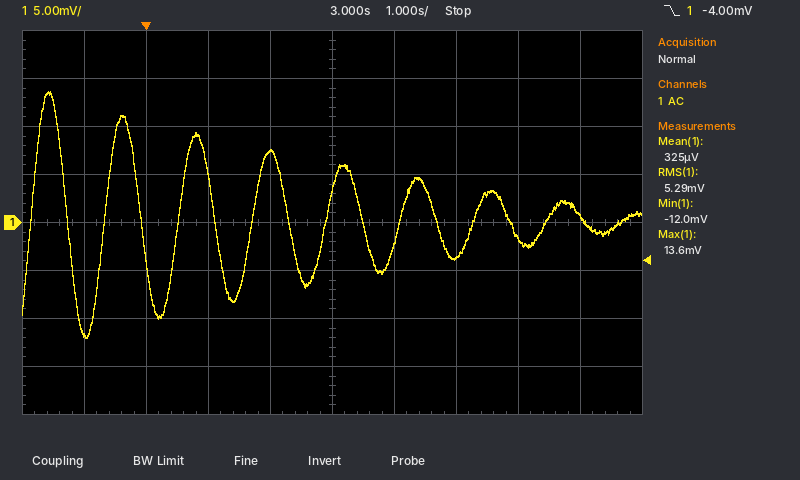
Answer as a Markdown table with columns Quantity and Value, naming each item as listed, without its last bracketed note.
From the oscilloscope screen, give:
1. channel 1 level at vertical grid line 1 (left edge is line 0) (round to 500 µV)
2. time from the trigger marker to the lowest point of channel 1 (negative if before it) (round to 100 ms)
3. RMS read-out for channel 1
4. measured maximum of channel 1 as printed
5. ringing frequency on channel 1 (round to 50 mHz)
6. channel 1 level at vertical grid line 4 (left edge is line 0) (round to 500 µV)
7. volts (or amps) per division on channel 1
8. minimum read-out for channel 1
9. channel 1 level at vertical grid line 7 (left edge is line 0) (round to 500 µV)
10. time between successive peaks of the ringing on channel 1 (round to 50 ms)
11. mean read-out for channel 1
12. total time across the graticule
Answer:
| Quantity | Value |
|---|---|
| channel 1 level at vertical grid line 1 (left edge is line 0) | -11.5 mV |
| time from the trigger marker to the lowest point of channel 1 (negative if before it) | -1.0 s |
| RMS read-out for channel 1 | 5.29 mV |
| measured maximum of channel 1 as printed | 13.6 mV |
| ringing frequency on channel 1 | 850 mHz |
| channel 1 level at vertical grid line 4 (left edge is line 0) | 7.5 mV |
| volts (or amps) per division on channel 1 | 5 mV |
| minimum read-out for channel 1 | -12.0 mV |
| channel 1 level at vertical grid line 7 (left edge is line 0) | -3.5 mV |
| time between successive peaks of the ringing on channel 1 | 1.20 s |
| mean read-out for channel 1 | 325 µV |
| total time across the graticule | 10 s |
